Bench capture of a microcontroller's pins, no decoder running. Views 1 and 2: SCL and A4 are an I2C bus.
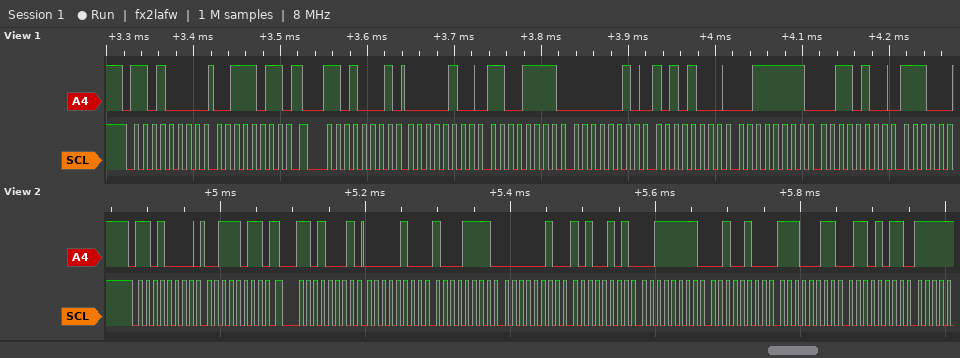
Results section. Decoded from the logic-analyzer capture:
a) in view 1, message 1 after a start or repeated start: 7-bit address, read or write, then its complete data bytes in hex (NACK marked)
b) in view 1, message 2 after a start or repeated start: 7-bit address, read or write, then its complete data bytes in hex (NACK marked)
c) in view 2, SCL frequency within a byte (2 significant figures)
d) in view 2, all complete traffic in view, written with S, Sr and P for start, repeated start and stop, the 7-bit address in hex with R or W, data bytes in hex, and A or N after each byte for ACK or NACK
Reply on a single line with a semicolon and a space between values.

0x68 write: 3B; 0x68 read: 04 CF 02 A8 3F 34; 100 kHz; S 68W A 3B A Sr 68R A 04 A 8F A 02 A A5 A 3F A 24 A E3 A 6B A
